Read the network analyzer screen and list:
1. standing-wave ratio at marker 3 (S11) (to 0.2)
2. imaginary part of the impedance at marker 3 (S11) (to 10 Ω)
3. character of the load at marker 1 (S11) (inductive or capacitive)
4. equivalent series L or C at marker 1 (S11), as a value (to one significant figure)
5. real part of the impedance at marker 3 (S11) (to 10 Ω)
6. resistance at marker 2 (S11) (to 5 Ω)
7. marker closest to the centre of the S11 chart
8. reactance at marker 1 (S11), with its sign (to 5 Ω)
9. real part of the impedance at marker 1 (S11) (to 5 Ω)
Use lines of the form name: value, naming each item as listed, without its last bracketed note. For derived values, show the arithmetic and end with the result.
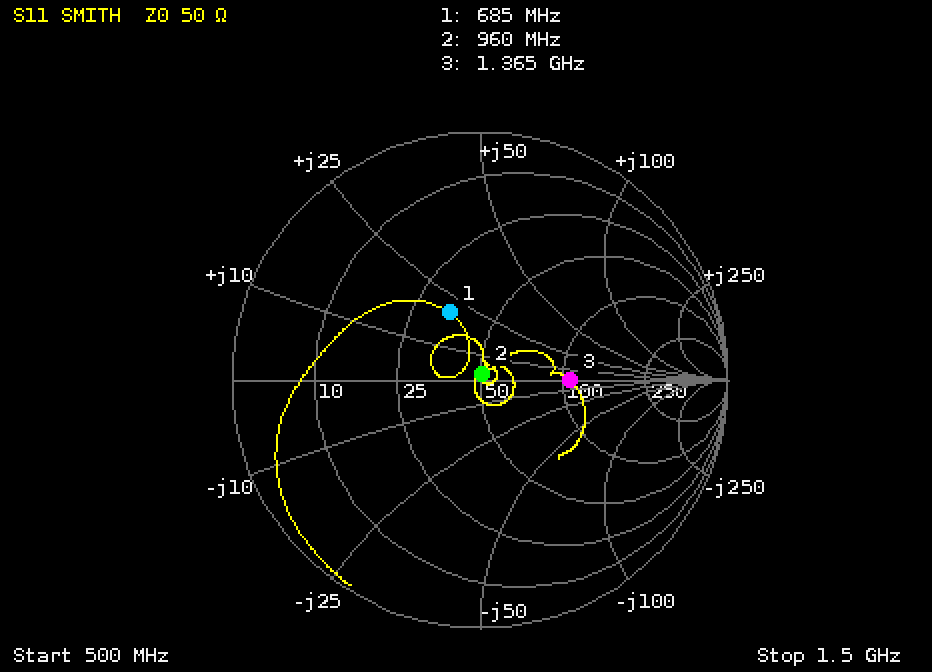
standing-wave ratio at marker 3 (S11): 2.2
imaginary part of the impedance at marker 3 (S11): 0 Ω
character of the load at marker 1 (S11): inductive
equivalent series L or C at marker 1 (S11), as a value: L = 20 Ω/(2π × 685 MHz) ≈ 5 nH
real part of the impedance at marker 3 (S11): 110 Ω
resistance at marker 2 (S11): 50 Ω
marker closest to the centre of the S11 chart: marker 2
reactance at marker 1 (S11), with its sign: +20 Ω
real part of the impedance at marker 1 (S11): 35 Ω
